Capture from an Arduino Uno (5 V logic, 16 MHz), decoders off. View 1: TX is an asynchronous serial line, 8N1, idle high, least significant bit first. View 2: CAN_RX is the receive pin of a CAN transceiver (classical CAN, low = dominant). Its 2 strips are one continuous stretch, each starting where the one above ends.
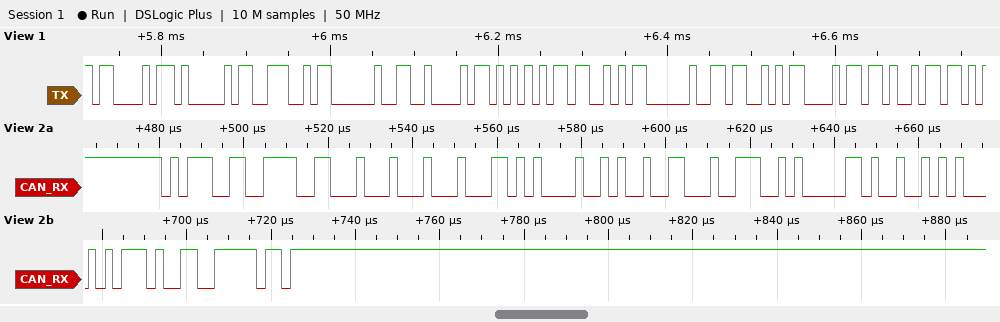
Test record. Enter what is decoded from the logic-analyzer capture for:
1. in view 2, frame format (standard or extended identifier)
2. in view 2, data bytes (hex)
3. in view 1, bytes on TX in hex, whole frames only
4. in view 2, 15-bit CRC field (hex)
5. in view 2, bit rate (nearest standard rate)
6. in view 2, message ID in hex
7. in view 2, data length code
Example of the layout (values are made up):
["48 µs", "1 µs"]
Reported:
["extended", "D4 25 26 27 28 29 2A 2B", "0x43 0x41 0x4E 0x20 0x42 0x55 0x53 0x20 0x53 0x68 0x69", "0x533F", "500 kbit/s", "0x17333111", "8"]
